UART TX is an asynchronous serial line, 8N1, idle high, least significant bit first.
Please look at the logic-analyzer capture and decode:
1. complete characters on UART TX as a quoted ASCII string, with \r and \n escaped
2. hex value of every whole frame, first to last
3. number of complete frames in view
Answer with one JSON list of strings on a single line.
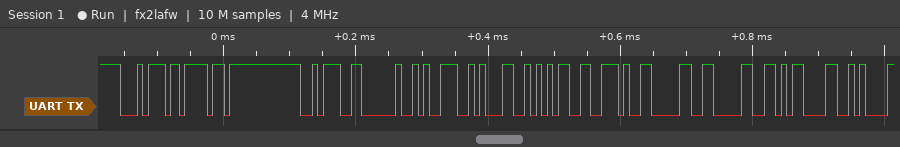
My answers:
["\"to: 915.00\\r\\n\"", "74 6F 3A 20 39 31 35 2E 30 30 0D 0A", "12"]
